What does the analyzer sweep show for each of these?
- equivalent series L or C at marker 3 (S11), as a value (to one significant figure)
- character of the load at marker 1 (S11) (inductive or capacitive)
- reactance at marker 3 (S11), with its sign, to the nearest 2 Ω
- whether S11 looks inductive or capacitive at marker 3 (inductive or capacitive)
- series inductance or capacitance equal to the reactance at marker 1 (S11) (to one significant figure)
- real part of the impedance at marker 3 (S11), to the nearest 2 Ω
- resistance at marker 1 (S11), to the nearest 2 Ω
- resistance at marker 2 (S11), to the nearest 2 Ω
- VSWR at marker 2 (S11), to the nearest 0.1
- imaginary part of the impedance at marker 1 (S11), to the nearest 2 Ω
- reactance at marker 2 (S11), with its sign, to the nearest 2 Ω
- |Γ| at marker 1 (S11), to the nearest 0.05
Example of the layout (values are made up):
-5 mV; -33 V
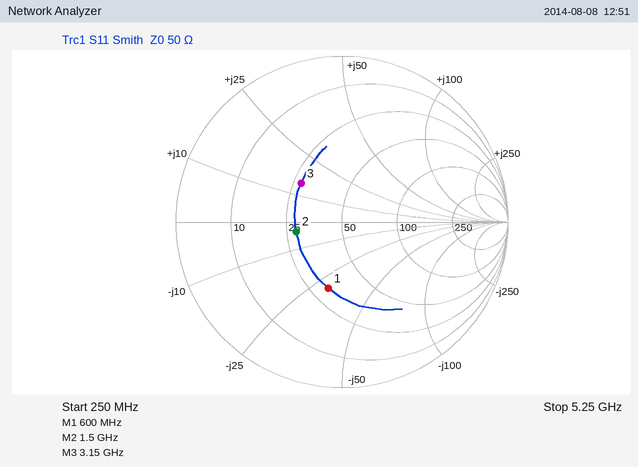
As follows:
700 pH; capacitive; +14 Ω; inductive; 9 pF; 28 Ω; 32 Ω; 28 Ω; 1.8; -30 Ω; -4 Ω; 0.40
